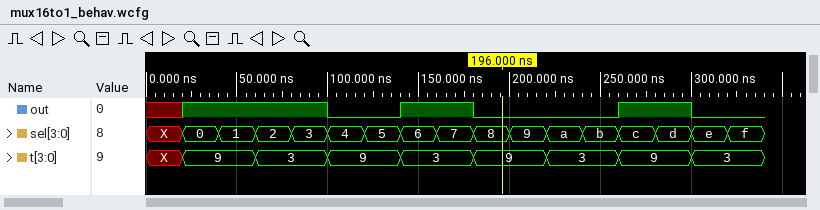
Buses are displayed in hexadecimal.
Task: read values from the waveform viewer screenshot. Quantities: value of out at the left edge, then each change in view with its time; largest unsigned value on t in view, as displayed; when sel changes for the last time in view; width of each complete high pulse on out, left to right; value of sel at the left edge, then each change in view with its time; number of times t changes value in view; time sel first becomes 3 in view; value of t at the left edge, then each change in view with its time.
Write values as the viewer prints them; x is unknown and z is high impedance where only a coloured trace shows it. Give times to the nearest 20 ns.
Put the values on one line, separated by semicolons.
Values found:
x, 1 at 20 ns, 0 at 100 ns, 1 at 140 ns, 0 at 180 ns, 1 at 260 ns, 0 at 300 ns; 9; 320 ns; 40 ns, 40 ns; X, 0 at 20 ns, 1 at 40 ns, 2 at 60 ns, 3 at 80 ns, 4 at 100 ns, 5 at 120 ns, 6 at 140 ns, 7 at 160 ns, 8 at 180 ns, 9 at 200 ns, a at 220 ns, b at 240 ns, c at 260 ns, d at 280 ns, e at 300 ns, f at 320 ns; 8; 80 ns; X, 9 at 20 ns, 3 at 60 ns, 9 at 100 ns, 3 at 140 ns, 9 at 180 ns, 3 at 220 ns, 9 at 260 ns, 3 at 300 ns
